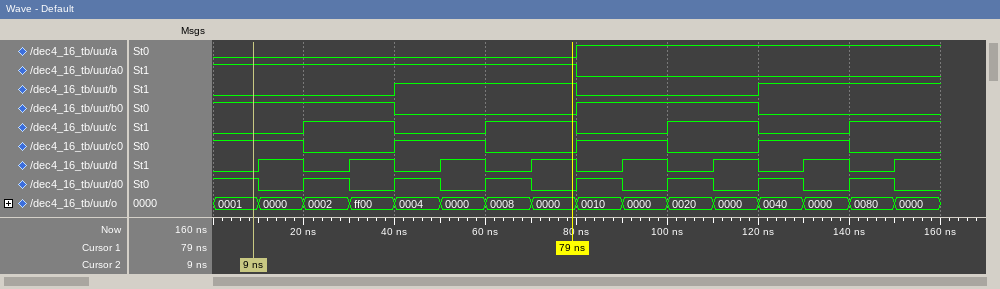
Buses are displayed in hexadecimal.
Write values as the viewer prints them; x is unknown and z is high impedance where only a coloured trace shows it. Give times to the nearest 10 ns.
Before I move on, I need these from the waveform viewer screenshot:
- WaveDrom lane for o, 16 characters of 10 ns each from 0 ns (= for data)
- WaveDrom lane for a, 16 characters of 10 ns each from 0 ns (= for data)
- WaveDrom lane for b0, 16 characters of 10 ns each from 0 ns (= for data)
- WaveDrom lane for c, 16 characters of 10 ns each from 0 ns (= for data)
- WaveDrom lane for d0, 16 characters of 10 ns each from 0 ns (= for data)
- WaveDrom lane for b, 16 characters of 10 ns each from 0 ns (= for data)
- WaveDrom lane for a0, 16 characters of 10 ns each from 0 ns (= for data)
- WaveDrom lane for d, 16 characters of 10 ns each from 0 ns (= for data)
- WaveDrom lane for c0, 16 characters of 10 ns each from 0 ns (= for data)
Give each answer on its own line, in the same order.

{name: 'o', wave: '================', data: '0001 0000 0002 ff00 0004 0000 0008 0000 0010 0000 0020 0000 0040 0000 0080 0000'}
{name: 'a', wave: '0.......1.......'}
{name: 'b0', wave: '1...0...1...0...'}
{name: 'c', wave: '0.1.0.1.0.1.0.1.'}
{name: 'd0', wave: '1010101010101010'}
{name: 'b', wave: '0...1...0...1...'}
{name: 'a0', wave: '1.......0.......'}
{name: 'd', wave: '0101010101010101'}
{name: 'c0', wave: '1.0.1.0.1.0.1.0.'}
